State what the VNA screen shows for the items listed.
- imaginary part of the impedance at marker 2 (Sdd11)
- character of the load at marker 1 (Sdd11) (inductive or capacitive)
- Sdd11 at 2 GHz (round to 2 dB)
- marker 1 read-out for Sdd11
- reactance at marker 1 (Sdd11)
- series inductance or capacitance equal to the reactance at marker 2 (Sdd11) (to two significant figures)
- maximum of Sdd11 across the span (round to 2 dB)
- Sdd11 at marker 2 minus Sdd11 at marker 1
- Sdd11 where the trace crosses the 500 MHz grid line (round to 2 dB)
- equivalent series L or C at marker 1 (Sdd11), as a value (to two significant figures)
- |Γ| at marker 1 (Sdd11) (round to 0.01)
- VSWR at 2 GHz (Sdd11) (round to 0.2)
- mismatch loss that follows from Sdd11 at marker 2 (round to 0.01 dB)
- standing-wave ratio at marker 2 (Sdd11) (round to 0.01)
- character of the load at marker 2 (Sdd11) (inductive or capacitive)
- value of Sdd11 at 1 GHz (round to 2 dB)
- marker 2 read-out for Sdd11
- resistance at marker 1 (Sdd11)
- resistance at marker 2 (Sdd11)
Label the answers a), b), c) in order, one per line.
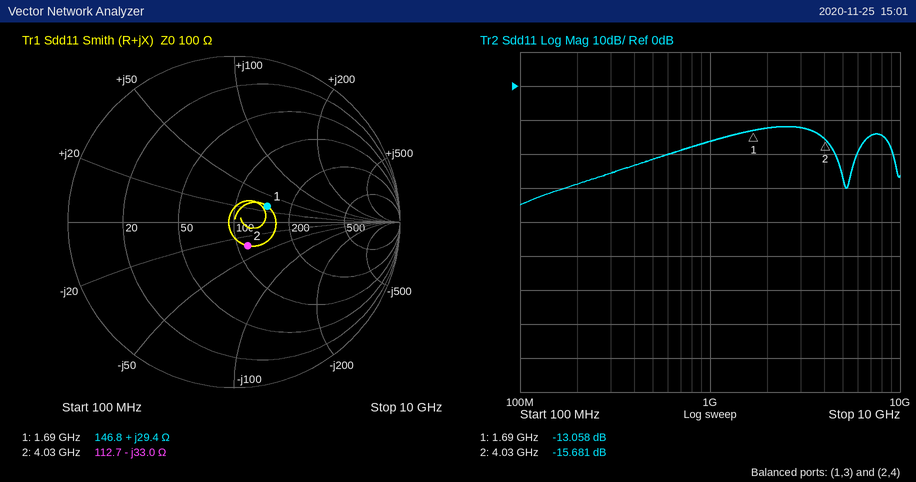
a) -33.0 Ω
b) inductive
c) -12 dB
d) -13.058 dB
e) +29.4 Ω
f) 1.2 pF
g) -12 dB
h) -2.623 dB
i) -22 dB
j) 2.8 nH
k) 0.22
l) 1.6
m) 0.12 dB
n) 1.39
o) capacitive
p) -16 dB
q) -15.681 dB
r) 146.8 Ω
s) 112.7 Ω
